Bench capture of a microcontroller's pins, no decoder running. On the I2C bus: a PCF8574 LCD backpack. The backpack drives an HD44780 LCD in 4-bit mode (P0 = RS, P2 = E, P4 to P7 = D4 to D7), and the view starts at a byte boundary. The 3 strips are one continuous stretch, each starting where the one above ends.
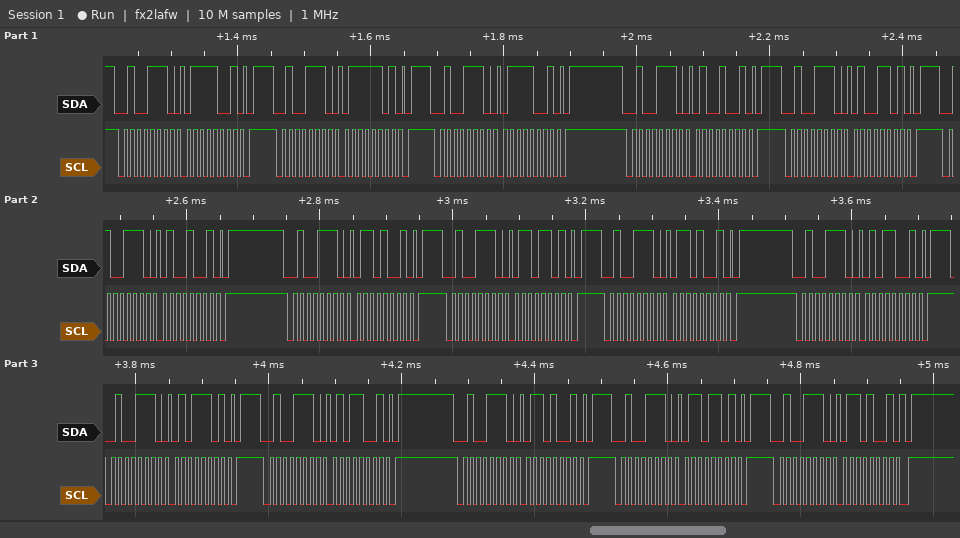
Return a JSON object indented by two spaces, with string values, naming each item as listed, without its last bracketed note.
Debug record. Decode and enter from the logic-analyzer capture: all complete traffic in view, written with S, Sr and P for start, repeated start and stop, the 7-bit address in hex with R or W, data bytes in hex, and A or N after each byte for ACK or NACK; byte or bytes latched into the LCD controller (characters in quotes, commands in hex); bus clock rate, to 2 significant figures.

{
  "all complete traffic in view, written with S, Sr and P for start, repeated start and stop, the 7-bit address in hex with R or W, data bytes in hex, and A or N after each byte for ACK or NACK": "S 27W A 79 A P S 27W A 7D A P S 27W A 79 A P S 27W A 49 A P S 27W A 4D A P S 27W A 49 A P S 27W A 69 A P S 27W A 6D A P S 27W A 69 A P S 27W A 59 A P S 27W A 5D A P S 27W A 59 A P S 27W A 69 A P S 27W A 6D A P S 27W A 69 A P",
  "byte or bytes latched into the LCD controller": "'t' 'e'",
  "bus clock rate, to 2 significant figures": "100 kHz"
}
